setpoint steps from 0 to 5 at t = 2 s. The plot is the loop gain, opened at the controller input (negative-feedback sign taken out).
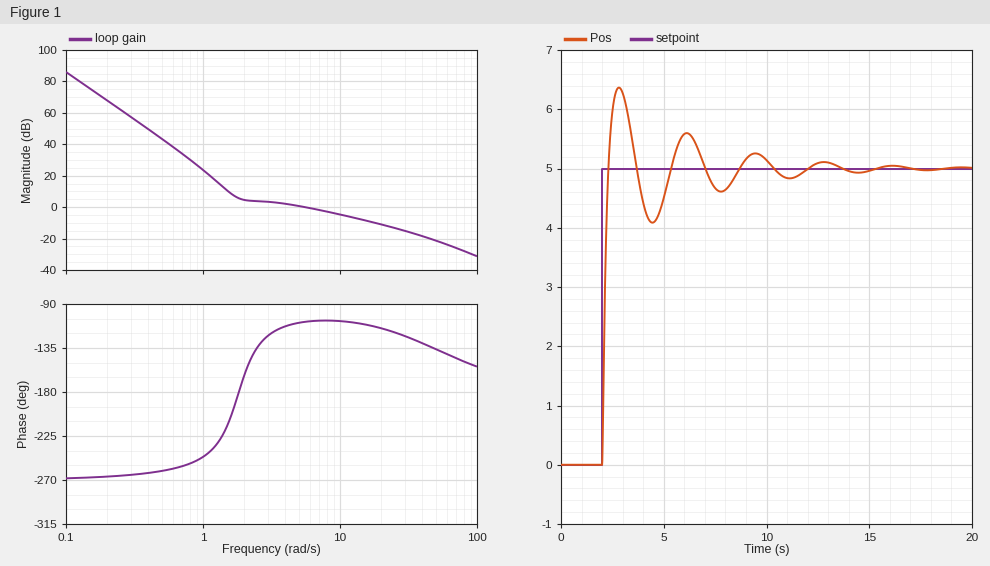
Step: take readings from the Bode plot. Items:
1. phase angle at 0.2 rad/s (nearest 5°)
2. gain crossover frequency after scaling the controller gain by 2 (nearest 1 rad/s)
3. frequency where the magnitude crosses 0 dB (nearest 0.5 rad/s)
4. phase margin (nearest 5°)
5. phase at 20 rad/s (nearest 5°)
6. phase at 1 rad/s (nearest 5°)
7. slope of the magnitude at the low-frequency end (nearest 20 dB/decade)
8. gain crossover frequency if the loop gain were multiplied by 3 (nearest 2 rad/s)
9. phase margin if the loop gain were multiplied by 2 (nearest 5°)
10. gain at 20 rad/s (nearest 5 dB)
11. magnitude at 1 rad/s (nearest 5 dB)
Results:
-265°
12 rad/s
5.5 rad/s
70°
-115°
-245°
-60 dB/decade
18 rad/s
70°
-10 dB
25 dB
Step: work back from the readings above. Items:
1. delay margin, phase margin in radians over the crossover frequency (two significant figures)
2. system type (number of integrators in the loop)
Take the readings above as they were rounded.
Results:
0.22 s
3
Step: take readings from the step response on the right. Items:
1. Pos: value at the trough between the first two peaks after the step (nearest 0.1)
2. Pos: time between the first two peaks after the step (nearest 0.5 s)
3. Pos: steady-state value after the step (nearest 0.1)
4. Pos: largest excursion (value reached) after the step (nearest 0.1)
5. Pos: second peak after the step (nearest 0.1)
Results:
4.1
3.5 s
5.0
6.4
5.6
